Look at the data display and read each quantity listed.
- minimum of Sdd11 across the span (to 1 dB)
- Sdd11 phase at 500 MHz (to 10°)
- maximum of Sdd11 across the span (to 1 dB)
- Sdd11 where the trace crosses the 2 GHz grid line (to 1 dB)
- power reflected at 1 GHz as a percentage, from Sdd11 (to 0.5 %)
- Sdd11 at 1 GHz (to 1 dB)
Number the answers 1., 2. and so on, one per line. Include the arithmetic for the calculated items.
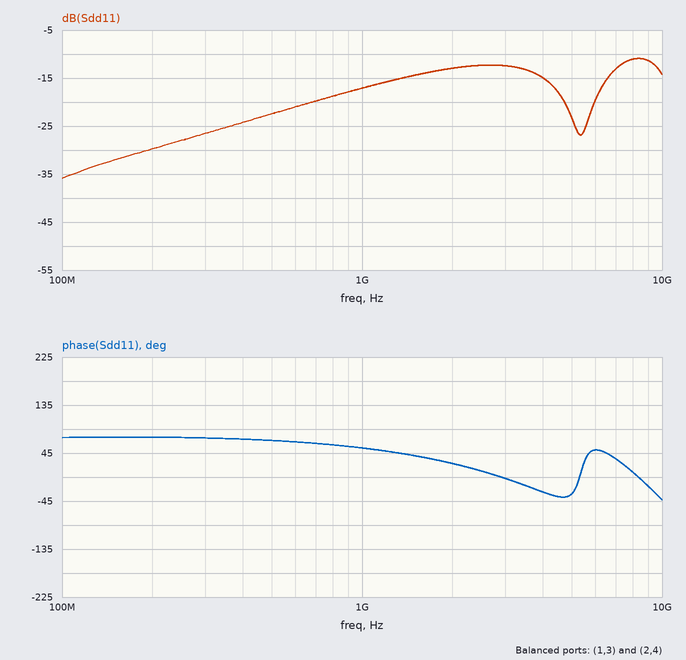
1. -36 dB
2. 70°
3. -11 dB
4. -13 dB
5. 10^(-17/10) ≈ 2.0 %
6. -17 dB
